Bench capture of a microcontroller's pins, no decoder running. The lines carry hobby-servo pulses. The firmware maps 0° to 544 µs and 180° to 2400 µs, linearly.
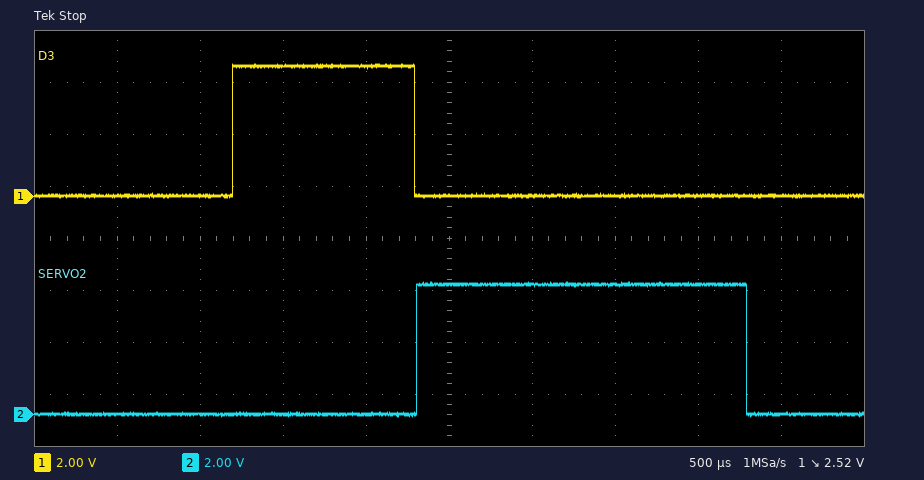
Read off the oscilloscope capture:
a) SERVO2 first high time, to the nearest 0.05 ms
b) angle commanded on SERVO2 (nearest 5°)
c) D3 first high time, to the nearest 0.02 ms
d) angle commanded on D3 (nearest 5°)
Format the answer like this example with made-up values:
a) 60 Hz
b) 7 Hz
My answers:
a) 2.00 ms
b) 140°
c) 1.10 ms
d) 55°
